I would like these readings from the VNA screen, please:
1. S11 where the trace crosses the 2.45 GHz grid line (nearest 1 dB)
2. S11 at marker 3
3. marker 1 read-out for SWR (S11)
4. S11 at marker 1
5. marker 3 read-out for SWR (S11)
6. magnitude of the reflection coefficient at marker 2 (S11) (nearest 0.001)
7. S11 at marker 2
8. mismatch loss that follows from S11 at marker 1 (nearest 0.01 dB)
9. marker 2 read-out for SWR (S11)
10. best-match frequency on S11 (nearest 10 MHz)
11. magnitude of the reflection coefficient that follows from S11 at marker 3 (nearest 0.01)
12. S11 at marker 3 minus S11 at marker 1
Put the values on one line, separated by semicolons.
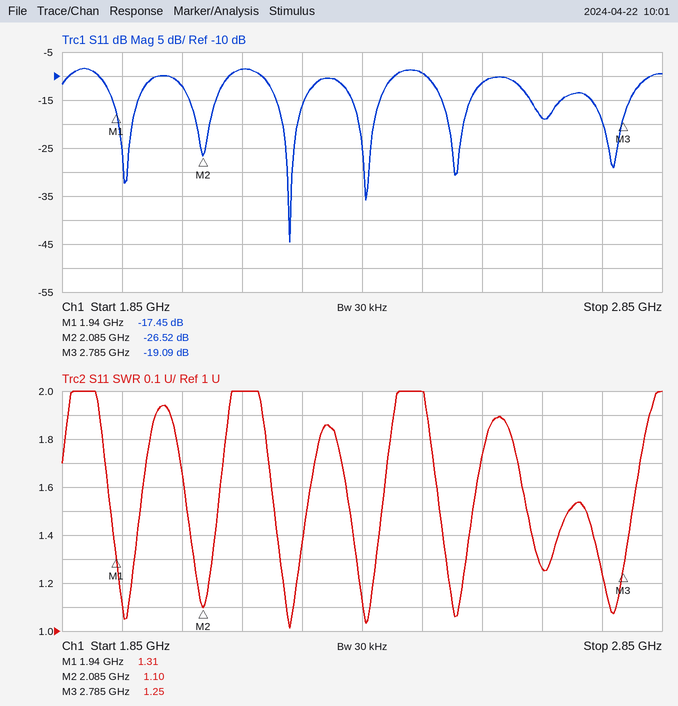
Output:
-9 dB; -19.09 dB; 1.31; -17.45 dB; 1.25; 0.047; -26.52 dB; 0.08 dB; 1.10; 2.23 GHz; 0.11; -1.64 dB
